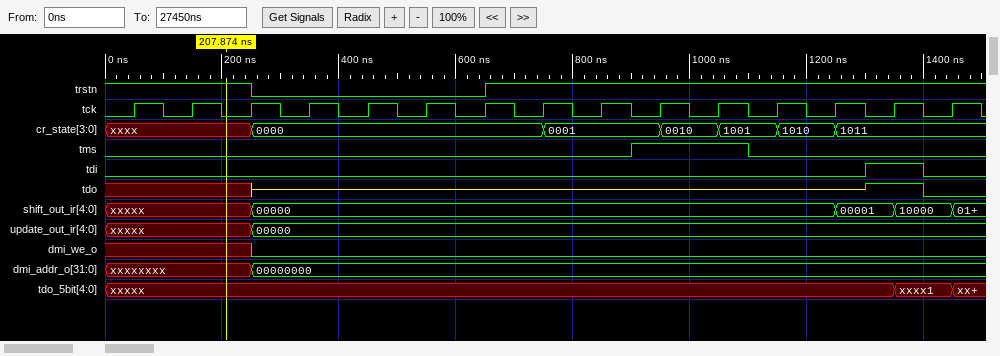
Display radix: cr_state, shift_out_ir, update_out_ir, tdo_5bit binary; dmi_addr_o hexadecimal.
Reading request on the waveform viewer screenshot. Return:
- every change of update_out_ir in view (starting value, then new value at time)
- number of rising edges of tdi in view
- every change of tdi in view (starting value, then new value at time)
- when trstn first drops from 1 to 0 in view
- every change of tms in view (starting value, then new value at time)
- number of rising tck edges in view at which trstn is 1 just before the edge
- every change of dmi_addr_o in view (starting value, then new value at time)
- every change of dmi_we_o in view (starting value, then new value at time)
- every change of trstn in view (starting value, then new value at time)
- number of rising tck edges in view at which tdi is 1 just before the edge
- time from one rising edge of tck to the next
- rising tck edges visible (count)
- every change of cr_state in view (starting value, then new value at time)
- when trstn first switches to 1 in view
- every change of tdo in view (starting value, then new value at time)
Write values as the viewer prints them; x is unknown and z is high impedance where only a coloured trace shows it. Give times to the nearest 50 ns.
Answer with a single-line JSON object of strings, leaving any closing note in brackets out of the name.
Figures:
{"every change of update_out_ir in view": "xxxxx, 00000 at 250 ns", "number of rising edges of tdi in view": "1", "every change of tdi in view": "0, 1 at 1300 ns, 0 at 1400 ns", "when trstn first drops from 1 to 0 in view": "250 ns", "every change of tms in view": "0, 1 at 900 ns, 0 at 1100 ns", "number of rising tck edges in view at which trstn is 1 just before the edge": "11", "every change of dmi_addr_o in view": "xxxxxxxx, 00000000 at 250 ns", "every change of dmi_we_o in view": "x, 0 at 250 ns", "every change of trstn in view": "1, 0 at 250 ns, 1 at 650 ns", "number of rising tck edges in view at which tdi is 1 just before the edge": "1", "time from one rising edge of tck to the next": "100 ns", "rising tck edges visible": "15", "every change of cr_state in view": "xxxx, 0000 at 250 ns, 0001 at 750 ns, 0010 at 950 ns, 1001 at 1050 ns, 1010 at 1150 ns, 1011 at 1250 ns", "when trstn first switches to 1 in view": "650 ns", "every change of tdo in view": "x, z at 250 ns, 1 at 1300 ns, 0 at 1400 ns"}
